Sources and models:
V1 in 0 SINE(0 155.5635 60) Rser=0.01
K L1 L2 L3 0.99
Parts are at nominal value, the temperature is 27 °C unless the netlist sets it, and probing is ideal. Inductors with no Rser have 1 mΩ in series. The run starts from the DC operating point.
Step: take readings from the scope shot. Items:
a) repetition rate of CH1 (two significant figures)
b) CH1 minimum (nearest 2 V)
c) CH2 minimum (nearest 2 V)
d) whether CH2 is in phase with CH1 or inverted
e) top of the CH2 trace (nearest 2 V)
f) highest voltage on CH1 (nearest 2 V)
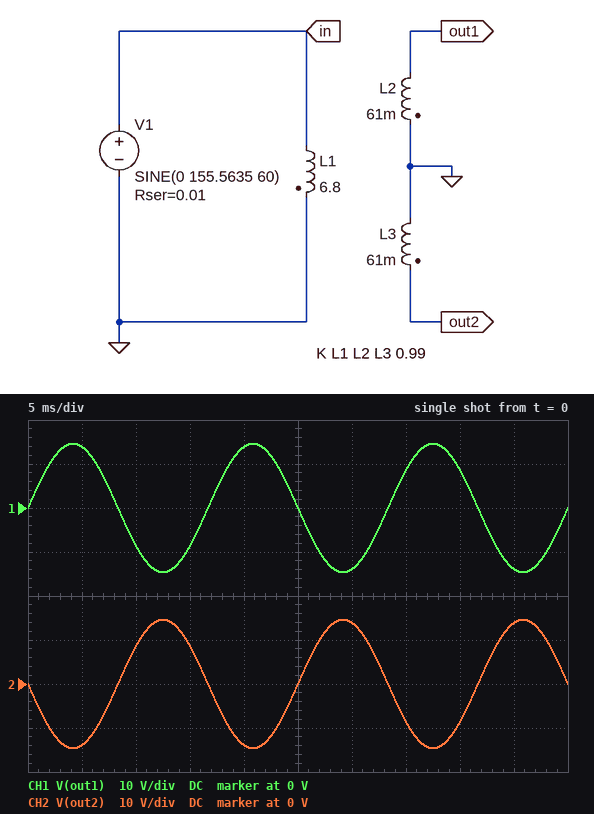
60 Hz
-14 V
-14 V
inverted
14 V
14 V
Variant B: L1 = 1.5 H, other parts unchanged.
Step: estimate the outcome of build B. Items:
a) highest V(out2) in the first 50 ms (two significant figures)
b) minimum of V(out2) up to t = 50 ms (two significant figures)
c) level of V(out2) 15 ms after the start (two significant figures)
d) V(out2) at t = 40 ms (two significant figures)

31 V
-31 V
18 V
-18 V
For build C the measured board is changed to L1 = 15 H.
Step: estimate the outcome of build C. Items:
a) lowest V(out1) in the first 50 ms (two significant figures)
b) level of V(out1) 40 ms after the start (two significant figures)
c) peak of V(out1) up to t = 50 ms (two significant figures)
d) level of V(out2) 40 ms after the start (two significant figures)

-9.8 V
5.8 V
9.8 V
-5.8 V
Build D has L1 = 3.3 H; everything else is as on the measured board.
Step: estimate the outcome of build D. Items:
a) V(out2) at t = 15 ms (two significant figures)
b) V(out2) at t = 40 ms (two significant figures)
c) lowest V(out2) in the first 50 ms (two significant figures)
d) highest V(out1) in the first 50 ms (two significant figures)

12 V
-12 V
-21 V
21 V
